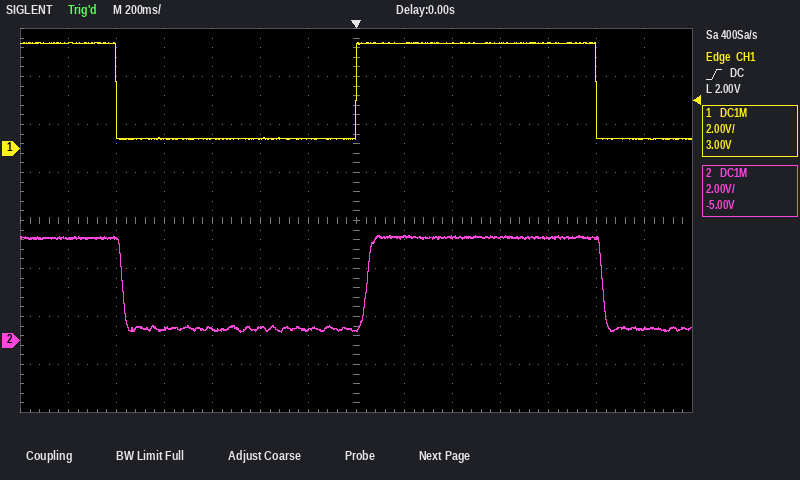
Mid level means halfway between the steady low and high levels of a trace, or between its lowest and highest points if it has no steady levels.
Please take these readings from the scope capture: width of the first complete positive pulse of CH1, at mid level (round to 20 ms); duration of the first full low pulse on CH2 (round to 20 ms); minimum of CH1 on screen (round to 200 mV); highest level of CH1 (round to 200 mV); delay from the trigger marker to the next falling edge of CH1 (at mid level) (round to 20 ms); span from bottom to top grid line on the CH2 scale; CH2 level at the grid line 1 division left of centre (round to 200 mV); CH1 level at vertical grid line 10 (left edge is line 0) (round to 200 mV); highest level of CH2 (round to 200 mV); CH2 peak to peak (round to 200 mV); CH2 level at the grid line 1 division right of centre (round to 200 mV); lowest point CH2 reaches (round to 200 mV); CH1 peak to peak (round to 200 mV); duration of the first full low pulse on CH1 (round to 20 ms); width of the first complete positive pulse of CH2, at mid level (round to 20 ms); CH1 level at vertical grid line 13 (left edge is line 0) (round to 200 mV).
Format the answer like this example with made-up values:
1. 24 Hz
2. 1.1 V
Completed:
1. 1.00 s
2. 1.02 s
3. 400 mV
4. 4.4 V
5. 1.00 s
6. 16 V
7. 400 mV
8. 4.4 V
9. 4.4 V
10. 4.0 V
11. 4.4 V
12. 400 mV
13. 4.0 V
14. 1.00 s
15. 980 ms
16. 400 mV
